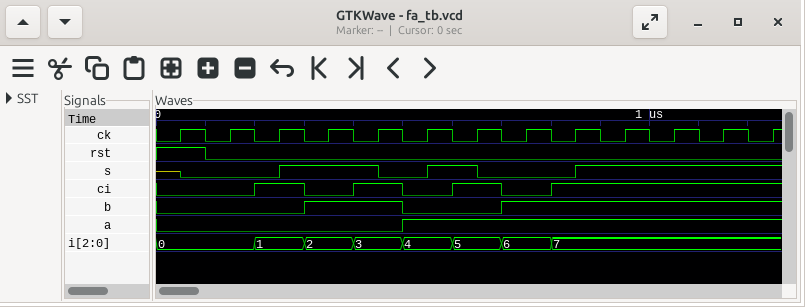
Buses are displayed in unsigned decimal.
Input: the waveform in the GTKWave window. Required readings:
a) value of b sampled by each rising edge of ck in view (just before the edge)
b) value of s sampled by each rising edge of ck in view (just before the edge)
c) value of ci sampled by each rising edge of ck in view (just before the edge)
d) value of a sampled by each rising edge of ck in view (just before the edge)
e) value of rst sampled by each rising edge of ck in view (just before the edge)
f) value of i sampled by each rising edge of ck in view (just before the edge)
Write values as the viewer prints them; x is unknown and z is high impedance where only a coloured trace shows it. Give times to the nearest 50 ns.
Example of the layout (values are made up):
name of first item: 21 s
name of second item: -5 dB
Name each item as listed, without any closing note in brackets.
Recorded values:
value of b sampled by each rising edge of ck in view: 0 0 0 1 1 0 0 1 1 1 1 1 1
value of s sampled by each rising edge of ck in view: z 0 0 1 1 0 1 0 0 1 1 1 1
value of ci sampled by each rising edge of ck in view: 0 0 1 0 1 0 1 0 1 1 1 1 1
value of a sampled by each rising edge of ck in view: 0 0 0 0 0 1 1 1 1 1 1 1 1
value of rst sampled by each rising edge of ck in view: 1 0 0 0 0 0 0 0 0 0 0 0 0
value of i sampled by each rising edge of ck in view: 0, 0, 1, 2, 3, 4, 5, 6, 7, 7, 7, 7, 7
